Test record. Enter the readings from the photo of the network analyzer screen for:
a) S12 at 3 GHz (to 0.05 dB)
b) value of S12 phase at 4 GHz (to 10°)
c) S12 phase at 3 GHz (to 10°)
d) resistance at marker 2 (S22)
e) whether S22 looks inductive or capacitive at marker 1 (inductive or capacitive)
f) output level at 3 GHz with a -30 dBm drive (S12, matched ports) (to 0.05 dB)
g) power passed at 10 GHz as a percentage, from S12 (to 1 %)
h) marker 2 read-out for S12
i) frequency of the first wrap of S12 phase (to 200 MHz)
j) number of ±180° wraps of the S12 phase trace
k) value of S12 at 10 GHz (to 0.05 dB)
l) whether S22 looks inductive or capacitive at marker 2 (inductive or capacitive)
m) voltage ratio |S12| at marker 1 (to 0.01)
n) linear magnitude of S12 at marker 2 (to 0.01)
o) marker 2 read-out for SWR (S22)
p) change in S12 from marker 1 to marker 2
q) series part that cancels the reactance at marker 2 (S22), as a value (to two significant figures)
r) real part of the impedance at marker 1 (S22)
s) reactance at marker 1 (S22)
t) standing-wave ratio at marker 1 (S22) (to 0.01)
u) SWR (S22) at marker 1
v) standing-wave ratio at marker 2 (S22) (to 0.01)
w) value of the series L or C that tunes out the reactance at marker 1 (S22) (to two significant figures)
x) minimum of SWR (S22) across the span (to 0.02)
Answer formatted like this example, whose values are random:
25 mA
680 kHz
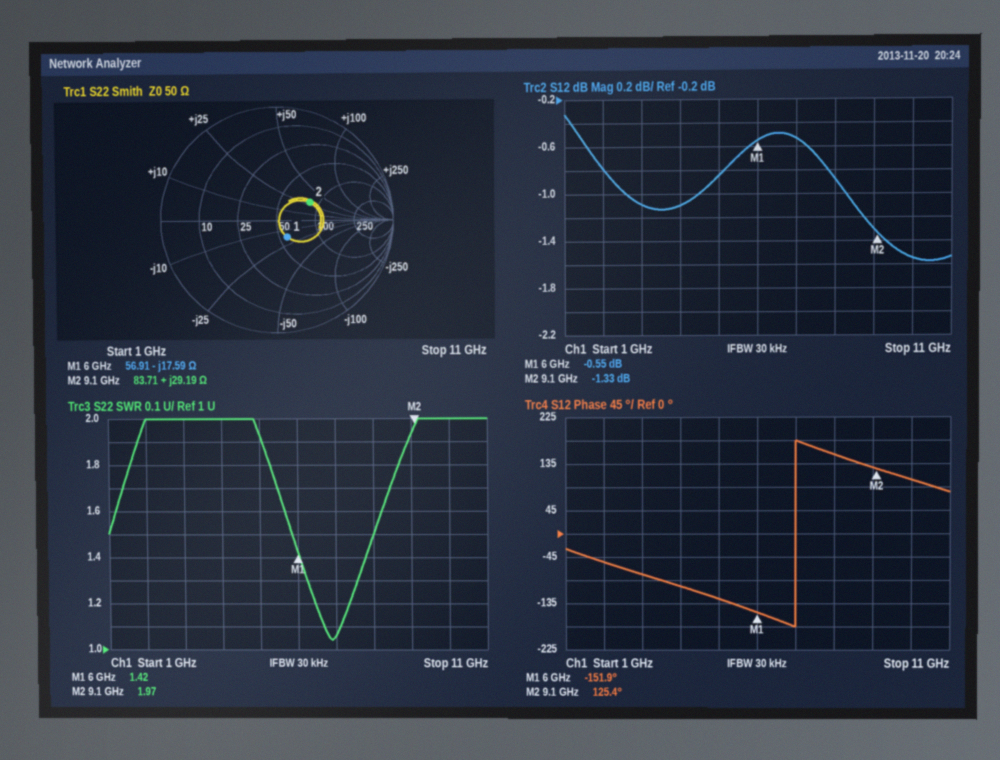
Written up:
-1.10 dB
-100°
-80°
83.71 Ω
capacitive
-31.10 dBm
70 %
-1.33 dB
7.0 GHz
1
-1.55 dB
inductive
0.94
0.86
1.97
-0.78 dB
600 fF
56.91 Ω
-17.59 Ω
1.42
1.42
1.97
470 pH
1.04
